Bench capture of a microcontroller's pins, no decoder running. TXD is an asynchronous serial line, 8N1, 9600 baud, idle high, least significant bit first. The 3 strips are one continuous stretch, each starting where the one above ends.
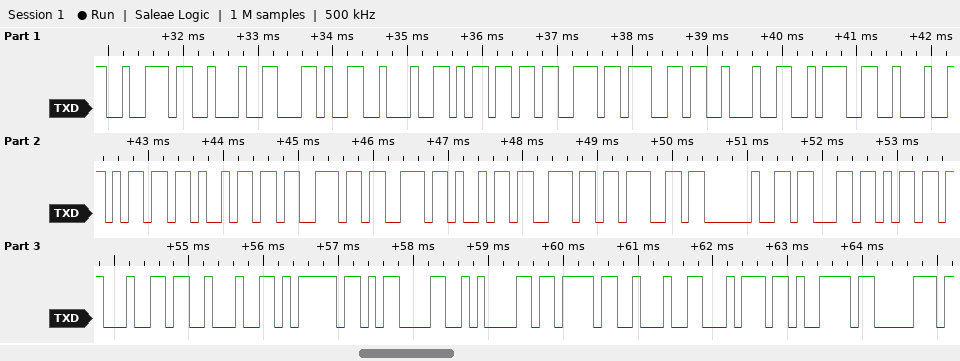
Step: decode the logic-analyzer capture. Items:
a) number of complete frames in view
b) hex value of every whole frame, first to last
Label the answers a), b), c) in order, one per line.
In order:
a) 30
b) 0x72 0x22 0x2C 0x22 0x6D 0x73 0x67 0x22 0x3A 0x22 0x6D 0x69 0x73 0x73 0x69 0x6E 0x67 0x20 0x63 0x6D 0x64 0x22 0x7D 0x0D 0x0A 0x7B 0x22 0x74 0x79 0x70
